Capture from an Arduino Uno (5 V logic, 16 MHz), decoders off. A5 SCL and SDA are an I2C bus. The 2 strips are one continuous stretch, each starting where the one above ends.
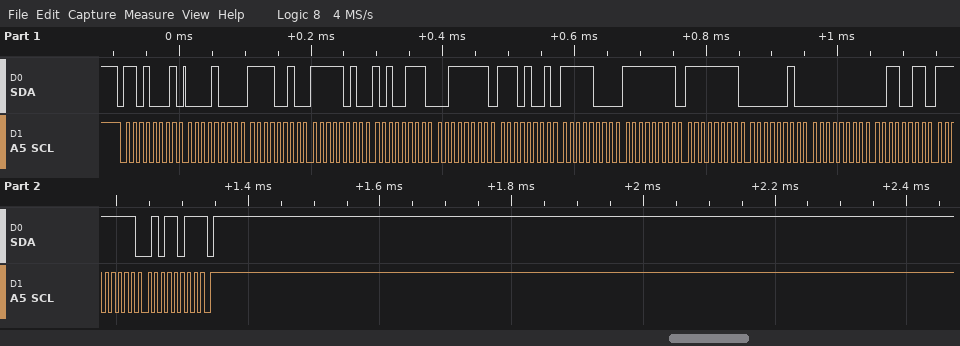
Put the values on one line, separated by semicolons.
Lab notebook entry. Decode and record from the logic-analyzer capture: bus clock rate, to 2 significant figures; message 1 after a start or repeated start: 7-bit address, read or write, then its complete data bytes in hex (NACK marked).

100 kHz; 0x68 read: 08 F2 FA A7 3F E9 F8 FF FF 02 00 33 FF 5B NACK
